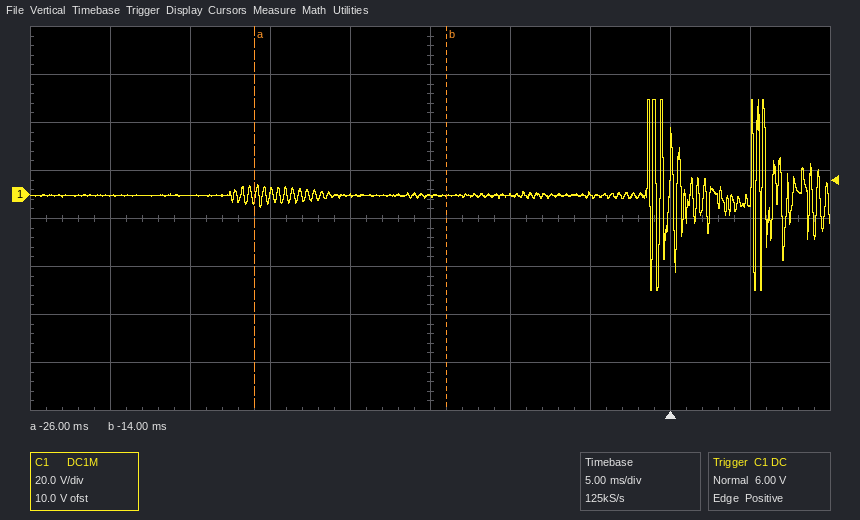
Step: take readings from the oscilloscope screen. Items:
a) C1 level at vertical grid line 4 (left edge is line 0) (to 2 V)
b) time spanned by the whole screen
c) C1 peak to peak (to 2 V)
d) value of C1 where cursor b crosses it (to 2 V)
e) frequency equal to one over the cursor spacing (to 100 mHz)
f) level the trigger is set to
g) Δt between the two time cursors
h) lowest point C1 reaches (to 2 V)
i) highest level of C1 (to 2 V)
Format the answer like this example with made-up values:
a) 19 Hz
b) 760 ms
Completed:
a) 0 V
b) 50 ms
c) 80 V
d) 0 V
e) 83.3 Hz
f) 6.00 V
g) 12.0 ms
h) -40 V
i) 40 V
